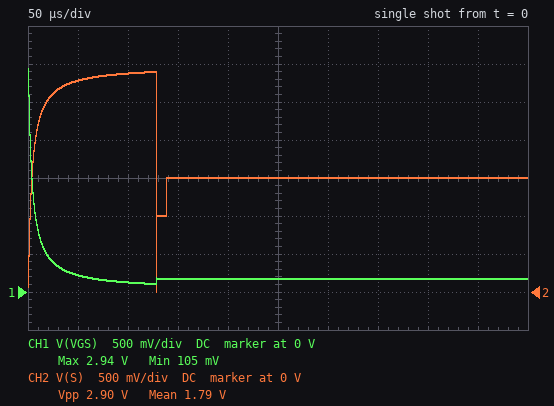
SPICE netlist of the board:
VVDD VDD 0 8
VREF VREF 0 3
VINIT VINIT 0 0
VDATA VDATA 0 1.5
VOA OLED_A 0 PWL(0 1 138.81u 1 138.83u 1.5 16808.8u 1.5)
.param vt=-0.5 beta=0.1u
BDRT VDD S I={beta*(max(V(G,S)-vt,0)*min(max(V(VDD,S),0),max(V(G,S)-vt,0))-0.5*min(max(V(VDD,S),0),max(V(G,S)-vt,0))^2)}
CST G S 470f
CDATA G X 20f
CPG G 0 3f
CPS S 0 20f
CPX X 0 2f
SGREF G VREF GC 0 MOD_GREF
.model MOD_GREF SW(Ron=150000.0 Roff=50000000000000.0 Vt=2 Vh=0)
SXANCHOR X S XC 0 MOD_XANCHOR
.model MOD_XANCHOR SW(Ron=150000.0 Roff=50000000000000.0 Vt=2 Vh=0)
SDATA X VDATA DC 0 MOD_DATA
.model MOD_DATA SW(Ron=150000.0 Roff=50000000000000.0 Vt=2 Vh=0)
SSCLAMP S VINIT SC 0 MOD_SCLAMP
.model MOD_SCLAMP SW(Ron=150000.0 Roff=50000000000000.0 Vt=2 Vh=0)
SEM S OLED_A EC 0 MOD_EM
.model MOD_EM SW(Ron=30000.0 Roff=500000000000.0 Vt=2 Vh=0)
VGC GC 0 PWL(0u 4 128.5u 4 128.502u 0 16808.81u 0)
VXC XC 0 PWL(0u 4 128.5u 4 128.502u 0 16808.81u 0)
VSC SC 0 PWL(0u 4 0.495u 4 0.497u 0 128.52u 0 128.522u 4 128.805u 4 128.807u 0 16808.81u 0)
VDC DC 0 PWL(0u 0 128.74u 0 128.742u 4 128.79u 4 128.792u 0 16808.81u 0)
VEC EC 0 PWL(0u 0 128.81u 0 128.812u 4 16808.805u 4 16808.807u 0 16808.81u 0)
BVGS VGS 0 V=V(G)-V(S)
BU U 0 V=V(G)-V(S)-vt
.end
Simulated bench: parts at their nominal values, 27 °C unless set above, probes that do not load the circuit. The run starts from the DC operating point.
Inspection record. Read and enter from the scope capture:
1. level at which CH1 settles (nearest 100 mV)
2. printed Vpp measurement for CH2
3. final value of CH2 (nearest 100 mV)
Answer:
200 mV
2.90 V
1.5 V
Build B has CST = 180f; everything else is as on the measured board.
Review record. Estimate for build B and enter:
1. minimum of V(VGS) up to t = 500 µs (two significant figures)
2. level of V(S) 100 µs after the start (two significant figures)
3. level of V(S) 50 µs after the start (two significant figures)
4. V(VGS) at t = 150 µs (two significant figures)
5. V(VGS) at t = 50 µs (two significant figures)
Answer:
61 mV
2.9 V
2.9 V
210 mV
110 mV
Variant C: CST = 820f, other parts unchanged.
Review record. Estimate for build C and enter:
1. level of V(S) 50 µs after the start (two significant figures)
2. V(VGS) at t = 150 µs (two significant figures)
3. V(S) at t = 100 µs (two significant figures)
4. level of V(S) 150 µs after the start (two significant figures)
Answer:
2.7 V
190 mV
2.8 V
1.5 V
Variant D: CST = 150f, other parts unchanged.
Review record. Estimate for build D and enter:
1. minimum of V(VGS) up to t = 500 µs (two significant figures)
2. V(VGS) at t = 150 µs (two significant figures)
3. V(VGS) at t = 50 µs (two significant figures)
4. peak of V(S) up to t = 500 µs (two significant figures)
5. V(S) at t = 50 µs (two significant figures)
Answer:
56 mV
230 mV
100 mV
2.9 V
2.9 V
